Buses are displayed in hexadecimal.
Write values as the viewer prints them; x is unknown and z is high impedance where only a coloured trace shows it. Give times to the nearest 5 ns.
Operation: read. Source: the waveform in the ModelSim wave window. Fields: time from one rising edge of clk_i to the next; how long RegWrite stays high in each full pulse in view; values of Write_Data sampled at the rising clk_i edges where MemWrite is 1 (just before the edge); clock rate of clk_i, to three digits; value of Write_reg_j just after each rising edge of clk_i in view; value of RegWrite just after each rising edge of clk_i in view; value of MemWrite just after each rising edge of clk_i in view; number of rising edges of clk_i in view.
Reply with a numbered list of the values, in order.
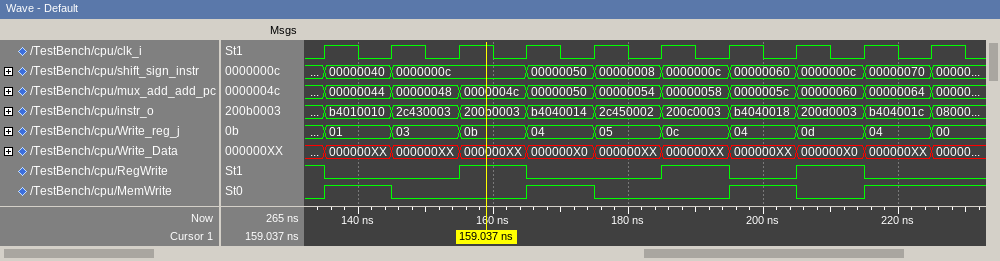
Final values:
1. 10 ns
2. 10 ns, 10 ns, 10 ns
3. 000000XX, 000000X0, 000000XX, 000000XX
4. 100 MHz
5. 01, 03, 0b, 04, 05, 0c, 04, 0d, 04, 00
6. 0 0 1 0 0 1 0 1 0 0
7. 1 0 0 1 0 0 1 0 1 1
8. 10
